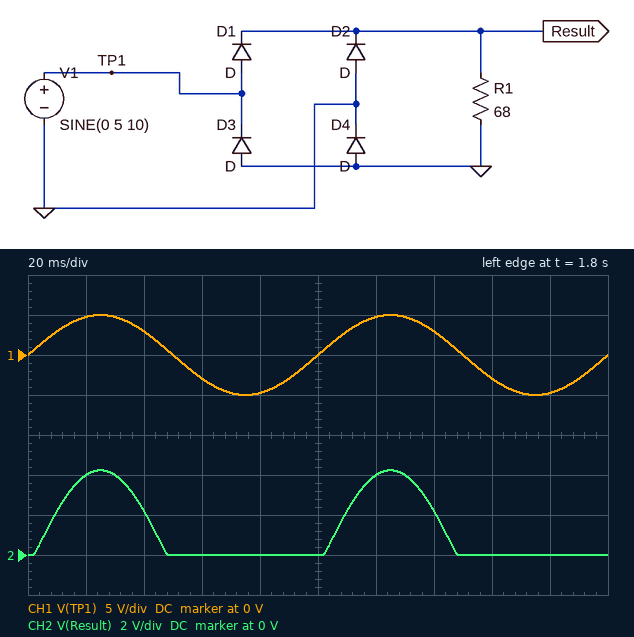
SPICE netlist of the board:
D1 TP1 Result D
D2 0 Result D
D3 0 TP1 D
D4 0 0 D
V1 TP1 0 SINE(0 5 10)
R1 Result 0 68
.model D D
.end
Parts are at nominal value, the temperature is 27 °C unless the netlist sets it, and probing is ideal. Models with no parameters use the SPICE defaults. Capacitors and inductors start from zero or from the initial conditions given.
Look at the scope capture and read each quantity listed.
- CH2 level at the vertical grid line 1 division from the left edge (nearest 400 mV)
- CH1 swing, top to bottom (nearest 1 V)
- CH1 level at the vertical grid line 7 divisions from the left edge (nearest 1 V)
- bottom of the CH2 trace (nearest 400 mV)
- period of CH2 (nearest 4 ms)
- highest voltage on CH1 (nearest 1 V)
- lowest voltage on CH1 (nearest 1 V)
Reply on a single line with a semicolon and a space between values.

4.0 V; 10 V; 3 V; 0 V; 100 ms; 5 V; -5 V
